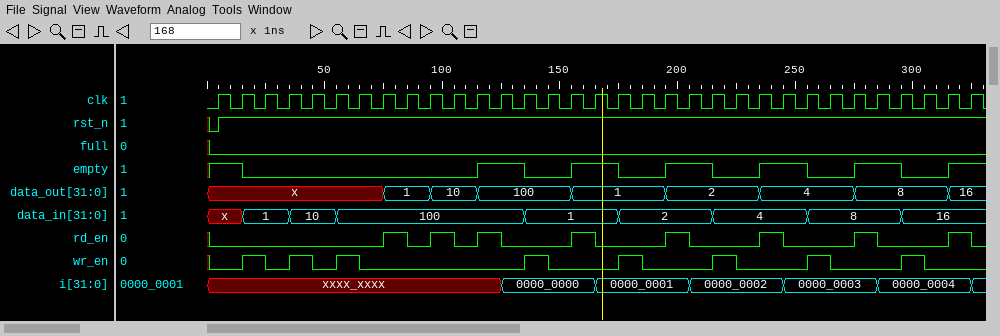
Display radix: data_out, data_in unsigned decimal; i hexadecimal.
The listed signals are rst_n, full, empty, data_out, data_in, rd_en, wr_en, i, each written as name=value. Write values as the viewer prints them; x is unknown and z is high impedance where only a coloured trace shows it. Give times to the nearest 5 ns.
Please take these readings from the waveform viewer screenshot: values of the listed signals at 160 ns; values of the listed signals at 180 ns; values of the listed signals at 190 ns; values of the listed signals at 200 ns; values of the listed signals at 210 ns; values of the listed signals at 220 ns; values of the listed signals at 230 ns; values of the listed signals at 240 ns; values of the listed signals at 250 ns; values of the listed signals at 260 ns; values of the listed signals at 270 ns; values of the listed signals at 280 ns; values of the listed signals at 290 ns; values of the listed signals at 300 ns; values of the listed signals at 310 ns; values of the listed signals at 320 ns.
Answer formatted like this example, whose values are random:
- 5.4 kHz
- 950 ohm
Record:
- rst_n=1, full=0, empty=1, data_out=1, data_in=1, rd_en=1, wr_en=0, i=0000_0000
- rst_n=1, full=0, empty=0, data_out=1, data_in=2, rd_en=0, wr_en=1, i=0000_0001
- rst_n=1, full=0, empty=0, data_out=1, data_in=2, rd_en=0, wr_en=0, i=0000_0001
- rst_n=1, full=0, empty=1, data_out=2, data_in=2, rd_en=1, wr_en=0, i=0000_0001
- rst_n=1, full=0, empty=1, data_out=2, data_in=2, rd_en=0, wr_en=0, i=0000_0002
- rst_n=1, full=0, empty=0, data_out=2, data_in=4, rd_en=0, wr_en=1, i=0000_0002
- rst_n=1, full=0, empty=0, data_out=2, data_in=4, rd_en=0, wr_en=0, i=0000_0002
- rst_n=1, full=0, empty=1, data_out=4, data_in=4, rd_en=1, wr_en=0, i=0000_0002
- rst_n=1, full=0, empty=1, data_out=4, data_in=4, rd_en=0, wr_en=0, i=0000_0003
- rst_n=1, full=0, empty=0, data_out=4, data_in=8, rd_en=0, wr_en=1, i=0000_0003
- rst_n=1, full=0, empty=0, data_out=4, data_in=8, rd_en=0, wr_en=0, i=0000_0003
- rst_n=1, full=0, empty=1, data_out=8, data_in=8, rd_en=1, wr_en=0, i=0000_0003
- rst_n=1, full=0, empty=1, data_out=8, data_in=8, rd_en=0, wr_en=0, i=0000_0004
- rst_n=1, full=0, empty=0, data_out=8, data_in=16, rd_en=0, wr_en=1, i=0000_0004
- rst_n=1, full=0, empty=0, data_out=8, data_in=16, rd_en=0, wr_en=0, i=0000_0004
- rst_n=1, full=0, empty=1, data_out=16, data_in=16, rd_en=1, wr_en=0, i=0000_0004
